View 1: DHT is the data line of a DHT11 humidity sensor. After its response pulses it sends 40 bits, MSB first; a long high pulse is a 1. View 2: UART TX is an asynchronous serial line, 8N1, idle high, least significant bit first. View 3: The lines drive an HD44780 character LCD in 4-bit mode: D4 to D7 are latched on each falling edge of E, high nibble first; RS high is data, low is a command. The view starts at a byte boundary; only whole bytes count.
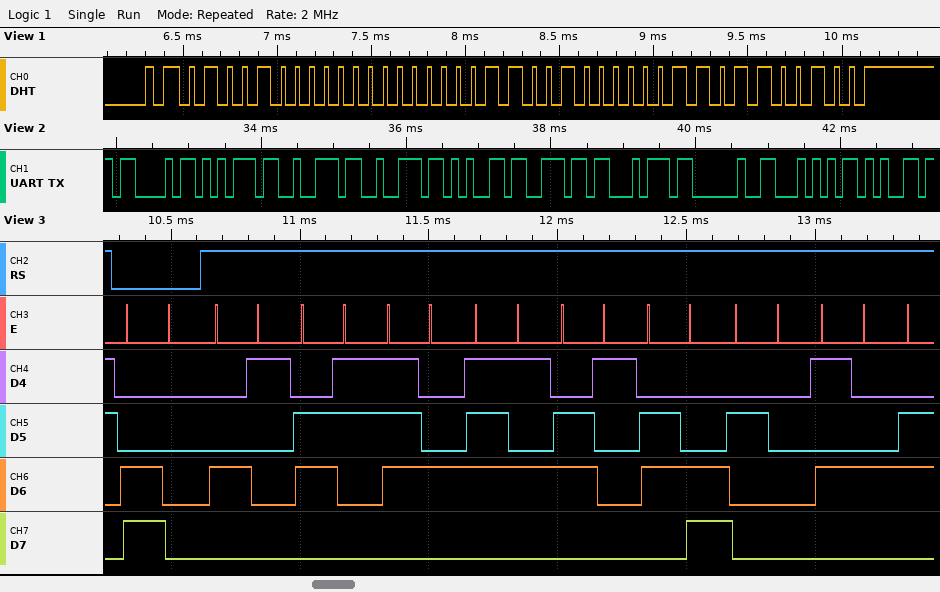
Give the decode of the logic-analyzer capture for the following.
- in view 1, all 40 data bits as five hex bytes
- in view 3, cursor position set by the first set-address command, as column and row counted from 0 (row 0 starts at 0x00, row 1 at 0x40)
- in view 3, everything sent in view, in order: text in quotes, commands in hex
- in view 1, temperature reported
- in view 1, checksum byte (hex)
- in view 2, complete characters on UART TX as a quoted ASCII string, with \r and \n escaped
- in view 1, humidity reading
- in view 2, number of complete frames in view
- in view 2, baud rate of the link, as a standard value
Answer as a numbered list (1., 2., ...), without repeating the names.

1. 48 00 19 03 64
2. column 0, row 1
3. 0xC0 "Actual T"
4. 25.3 °C
5. 0x64
6. "Current Te"
7. 72 %
8. 10
9. 9600 baud
